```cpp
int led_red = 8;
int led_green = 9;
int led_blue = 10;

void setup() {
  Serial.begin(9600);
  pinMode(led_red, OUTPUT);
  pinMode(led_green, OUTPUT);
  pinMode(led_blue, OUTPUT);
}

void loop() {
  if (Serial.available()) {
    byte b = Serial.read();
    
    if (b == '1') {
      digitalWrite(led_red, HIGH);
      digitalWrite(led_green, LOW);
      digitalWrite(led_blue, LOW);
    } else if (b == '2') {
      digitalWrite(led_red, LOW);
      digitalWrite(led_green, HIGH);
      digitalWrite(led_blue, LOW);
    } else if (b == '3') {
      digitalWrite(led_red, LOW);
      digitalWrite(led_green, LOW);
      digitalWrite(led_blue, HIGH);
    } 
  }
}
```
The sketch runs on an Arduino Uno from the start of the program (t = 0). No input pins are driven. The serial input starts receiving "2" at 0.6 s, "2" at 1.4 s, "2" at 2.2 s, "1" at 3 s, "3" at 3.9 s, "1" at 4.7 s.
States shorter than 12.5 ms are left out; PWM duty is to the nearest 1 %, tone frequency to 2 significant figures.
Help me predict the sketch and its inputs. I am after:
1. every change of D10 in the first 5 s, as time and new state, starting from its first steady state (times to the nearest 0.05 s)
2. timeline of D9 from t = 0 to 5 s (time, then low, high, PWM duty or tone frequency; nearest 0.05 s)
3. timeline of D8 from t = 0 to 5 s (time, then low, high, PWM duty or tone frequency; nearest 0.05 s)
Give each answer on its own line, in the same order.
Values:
0 s low; 3.9 s high; 4.7 s low
0 s low; 0.6 s high; 3 s low
0 s low; 3 s high; 3.9 s low; 4.7 s high
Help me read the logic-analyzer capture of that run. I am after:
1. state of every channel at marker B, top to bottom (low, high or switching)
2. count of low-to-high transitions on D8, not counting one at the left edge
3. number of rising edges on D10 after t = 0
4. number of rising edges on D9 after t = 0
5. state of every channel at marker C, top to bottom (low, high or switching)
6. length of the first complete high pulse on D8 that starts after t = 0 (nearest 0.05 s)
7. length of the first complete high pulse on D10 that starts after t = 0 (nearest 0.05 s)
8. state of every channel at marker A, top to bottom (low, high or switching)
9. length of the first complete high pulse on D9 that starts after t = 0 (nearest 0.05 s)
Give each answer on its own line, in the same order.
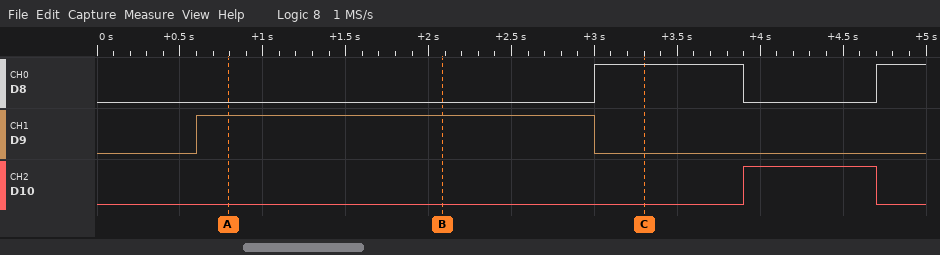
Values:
D8 low, D9 high, D10 low
2
1
1
D8 high, D9 low, D10 low
0.90 s
0.80 s
D8 low, D9 high, D10 low
2.40 s
